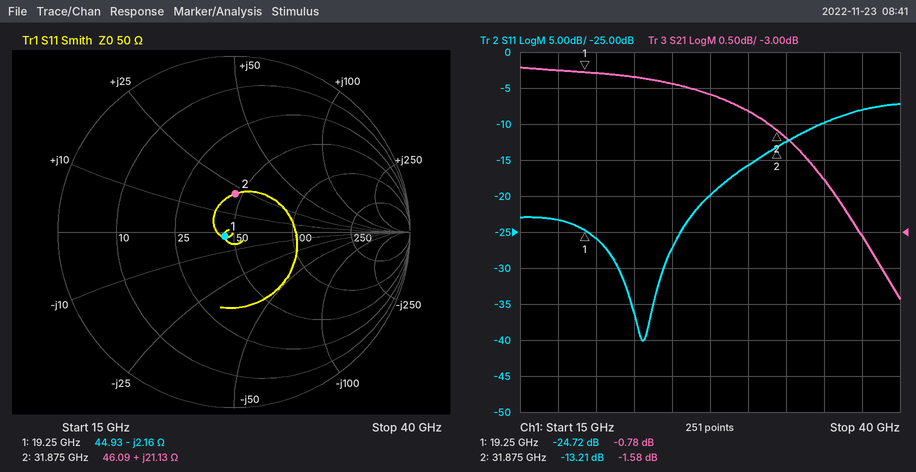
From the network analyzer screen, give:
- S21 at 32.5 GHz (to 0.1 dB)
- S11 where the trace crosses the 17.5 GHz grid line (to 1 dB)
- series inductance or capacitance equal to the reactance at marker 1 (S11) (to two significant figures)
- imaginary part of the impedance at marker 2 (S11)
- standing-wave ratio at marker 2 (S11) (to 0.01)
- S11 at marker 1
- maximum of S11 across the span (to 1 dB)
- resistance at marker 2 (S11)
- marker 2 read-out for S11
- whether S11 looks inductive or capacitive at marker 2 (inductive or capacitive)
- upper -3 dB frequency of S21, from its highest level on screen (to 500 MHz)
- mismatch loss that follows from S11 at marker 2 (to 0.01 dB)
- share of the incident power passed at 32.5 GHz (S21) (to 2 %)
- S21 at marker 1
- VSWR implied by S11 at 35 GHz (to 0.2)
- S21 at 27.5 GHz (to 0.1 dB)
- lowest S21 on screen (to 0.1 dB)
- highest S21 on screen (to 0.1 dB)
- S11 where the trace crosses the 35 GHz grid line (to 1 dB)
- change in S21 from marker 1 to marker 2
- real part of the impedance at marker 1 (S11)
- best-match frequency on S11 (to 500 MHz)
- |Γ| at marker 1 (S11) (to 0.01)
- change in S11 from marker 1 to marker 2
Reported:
-1.7 dB
-23 dB
3.8 pF
+21.13 Ω
1.56
-24.72 dB
-7 dB
46.09 Ω
-13.21 dB
inductive
39.5 GHz
0.21 dB
68 %
-0.78 dB
2.0
-1.1 dB
-3.9 dB
-0.7 dB
-10 dB
-0.80 dB
44.93 Ω
23.0 GHz
0.06
11.51 dB
